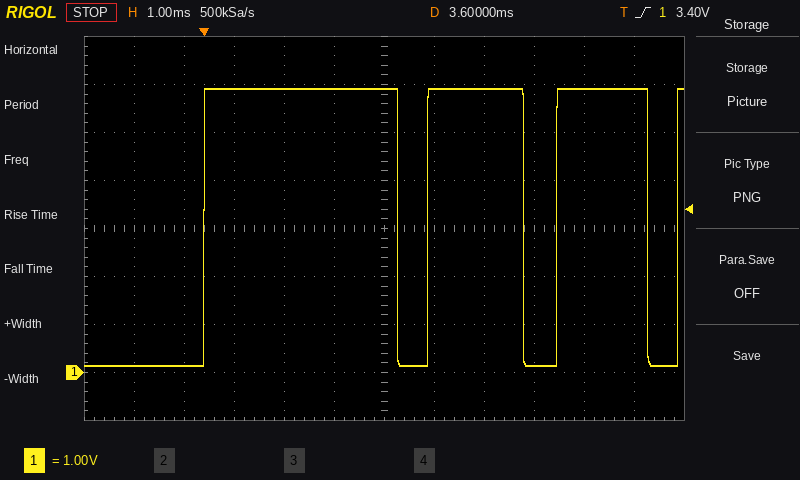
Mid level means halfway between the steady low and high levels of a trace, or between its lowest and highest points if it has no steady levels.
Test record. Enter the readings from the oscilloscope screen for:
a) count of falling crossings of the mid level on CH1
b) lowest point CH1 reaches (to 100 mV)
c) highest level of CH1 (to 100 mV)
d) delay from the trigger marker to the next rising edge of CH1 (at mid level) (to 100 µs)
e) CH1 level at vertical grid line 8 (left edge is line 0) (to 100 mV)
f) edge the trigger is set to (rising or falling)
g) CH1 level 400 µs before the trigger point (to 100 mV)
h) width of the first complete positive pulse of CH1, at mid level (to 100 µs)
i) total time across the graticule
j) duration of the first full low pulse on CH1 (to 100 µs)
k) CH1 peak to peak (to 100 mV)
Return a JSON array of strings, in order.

["3", "100 mV", "5.9 V", "4.5 ms", "5.9 V", "rising", "100 mV", "3.9 ms", "12 ms", "600 µs", "5.8 V"]
